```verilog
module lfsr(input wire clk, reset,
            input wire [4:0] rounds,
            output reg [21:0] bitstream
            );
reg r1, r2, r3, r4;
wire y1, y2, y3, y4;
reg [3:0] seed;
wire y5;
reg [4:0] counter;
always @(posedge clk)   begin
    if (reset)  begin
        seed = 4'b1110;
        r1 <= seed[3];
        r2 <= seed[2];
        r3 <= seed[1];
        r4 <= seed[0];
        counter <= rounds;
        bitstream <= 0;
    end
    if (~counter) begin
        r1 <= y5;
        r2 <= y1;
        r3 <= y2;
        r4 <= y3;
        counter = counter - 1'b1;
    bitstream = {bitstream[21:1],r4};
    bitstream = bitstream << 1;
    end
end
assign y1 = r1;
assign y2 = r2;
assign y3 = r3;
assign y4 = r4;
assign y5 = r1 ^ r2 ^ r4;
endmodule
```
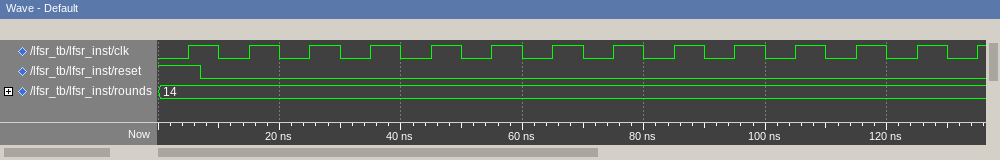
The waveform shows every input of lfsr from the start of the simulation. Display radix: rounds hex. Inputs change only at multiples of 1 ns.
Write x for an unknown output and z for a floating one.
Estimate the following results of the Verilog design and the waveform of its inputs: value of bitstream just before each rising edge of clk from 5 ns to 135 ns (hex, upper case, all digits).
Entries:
x, 000000, 000000, 000002, 000006, 00000E, 00001C, 000038, 000072, 0000E4, 0001CA, 000396, 00072E, 000E5C
